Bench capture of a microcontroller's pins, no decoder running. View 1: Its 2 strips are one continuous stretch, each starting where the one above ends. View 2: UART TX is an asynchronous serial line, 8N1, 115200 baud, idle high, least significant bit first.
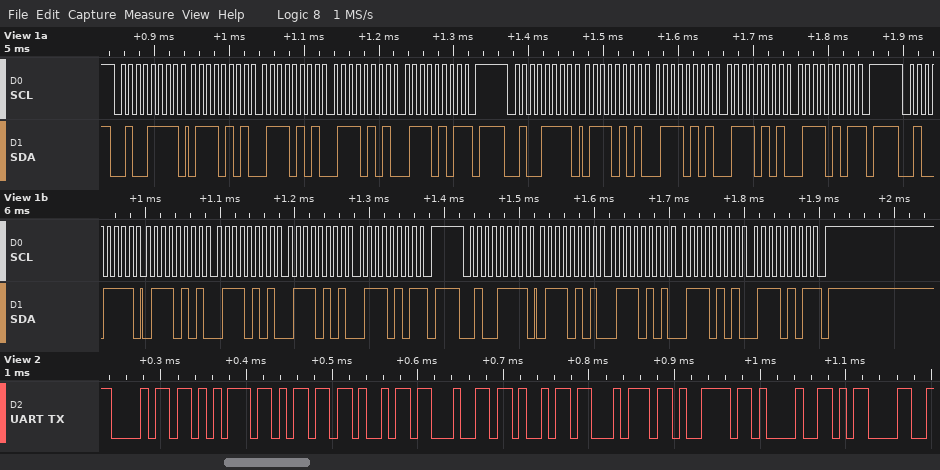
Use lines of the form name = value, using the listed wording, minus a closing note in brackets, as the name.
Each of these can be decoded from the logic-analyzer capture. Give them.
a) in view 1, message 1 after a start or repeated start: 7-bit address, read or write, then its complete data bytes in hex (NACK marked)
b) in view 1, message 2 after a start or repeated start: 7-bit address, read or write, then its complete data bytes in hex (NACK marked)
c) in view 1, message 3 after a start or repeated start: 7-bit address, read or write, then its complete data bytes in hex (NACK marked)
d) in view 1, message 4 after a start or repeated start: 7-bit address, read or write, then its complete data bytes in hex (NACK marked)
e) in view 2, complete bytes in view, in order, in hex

in view 1, message 1 after a start or repeated start: 7-bit address, read or write, then its complete data bytes in hex = 0x27 read: 75 75 75 75 NACK
in view 1, message 2 after a start or repeated start: 7-bit address, read or write, then its complete data bytes in hex = 0x27 read: 75 75 75 75 NACK
in view 1, message 3 after a start or repeated start: 7-bit address, read or write, then its complete data bytes in hex = 0x27 read: 75 75 75 75 NACK
in view 1, message 4 after a start or repeated start: 7-bit address, read or write, then its complete data bytes in hex = 0x27 read: 75 75 75 75 NACK
in view 2, complete bytes in view, in order, in hex = 0x68 0x75 0x6D 0x69 0x64 0x69 0x74 0x79 0x21 0x0D
